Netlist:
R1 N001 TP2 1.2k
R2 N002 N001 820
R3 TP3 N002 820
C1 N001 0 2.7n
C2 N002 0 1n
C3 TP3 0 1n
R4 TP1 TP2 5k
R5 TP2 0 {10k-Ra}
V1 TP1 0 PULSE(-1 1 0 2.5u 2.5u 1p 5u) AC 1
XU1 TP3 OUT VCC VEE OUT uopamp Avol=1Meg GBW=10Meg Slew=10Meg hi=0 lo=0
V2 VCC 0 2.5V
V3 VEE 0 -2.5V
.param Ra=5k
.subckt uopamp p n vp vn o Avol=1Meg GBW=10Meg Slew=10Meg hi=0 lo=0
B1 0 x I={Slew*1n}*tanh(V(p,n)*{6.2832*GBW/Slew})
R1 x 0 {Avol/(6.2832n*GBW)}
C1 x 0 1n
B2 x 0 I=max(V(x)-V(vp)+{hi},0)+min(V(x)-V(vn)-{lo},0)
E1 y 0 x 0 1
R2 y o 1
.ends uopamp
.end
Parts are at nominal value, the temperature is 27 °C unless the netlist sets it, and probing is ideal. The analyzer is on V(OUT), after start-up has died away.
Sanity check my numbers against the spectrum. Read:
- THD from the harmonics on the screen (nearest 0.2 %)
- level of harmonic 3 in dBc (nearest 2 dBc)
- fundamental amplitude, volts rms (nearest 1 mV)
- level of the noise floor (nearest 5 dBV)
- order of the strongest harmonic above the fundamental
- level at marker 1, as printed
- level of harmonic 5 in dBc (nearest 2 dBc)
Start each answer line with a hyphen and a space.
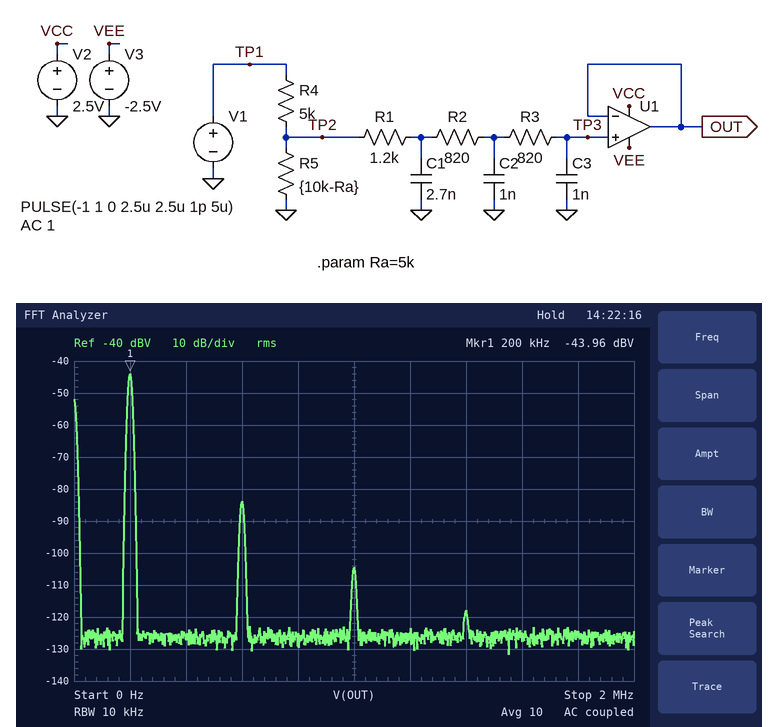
- 1.0 %
- -40 dBc
- 6 mV
- -125 dBV
- 3
- -43.96 dBV
- -60 dBc
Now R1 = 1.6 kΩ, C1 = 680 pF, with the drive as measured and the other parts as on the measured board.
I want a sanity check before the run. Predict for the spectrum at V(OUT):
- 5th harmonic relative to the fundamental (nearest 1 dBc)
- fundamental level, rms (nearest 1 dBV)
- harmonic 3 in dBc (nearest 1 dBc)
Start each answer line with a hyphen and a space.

- -57 dBc
- -37 dBV
- -37 dBc
